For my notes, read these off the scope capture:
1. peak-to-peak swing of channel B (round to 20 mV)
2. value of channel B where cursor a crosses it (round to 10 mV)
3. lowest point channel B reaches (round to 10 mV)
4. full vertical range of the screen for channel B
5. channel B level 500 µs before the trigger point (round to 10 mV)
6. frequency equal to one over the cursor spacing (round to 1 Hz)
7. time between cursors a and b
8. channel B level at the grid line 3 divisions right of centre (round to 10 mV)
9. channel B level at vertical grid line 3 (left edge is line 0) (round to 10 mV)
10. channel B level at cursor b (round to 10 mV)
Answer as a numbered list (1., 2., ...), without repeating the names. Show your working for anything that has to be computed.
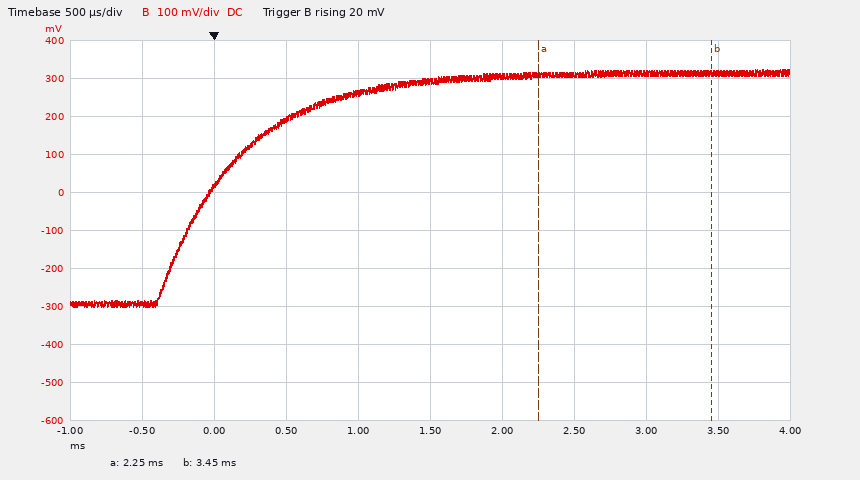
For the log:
1. 620 mV
2. 310 mV
3. -300 mV
4. 1 V
5. -290 mV
6. 1 / 1.20 ms ≈ 833 Hz
7. 3.45 ms − (2.25 ms) = 1.20 ms
8. 310 mV
9. 190 mV
10. 310 mV
